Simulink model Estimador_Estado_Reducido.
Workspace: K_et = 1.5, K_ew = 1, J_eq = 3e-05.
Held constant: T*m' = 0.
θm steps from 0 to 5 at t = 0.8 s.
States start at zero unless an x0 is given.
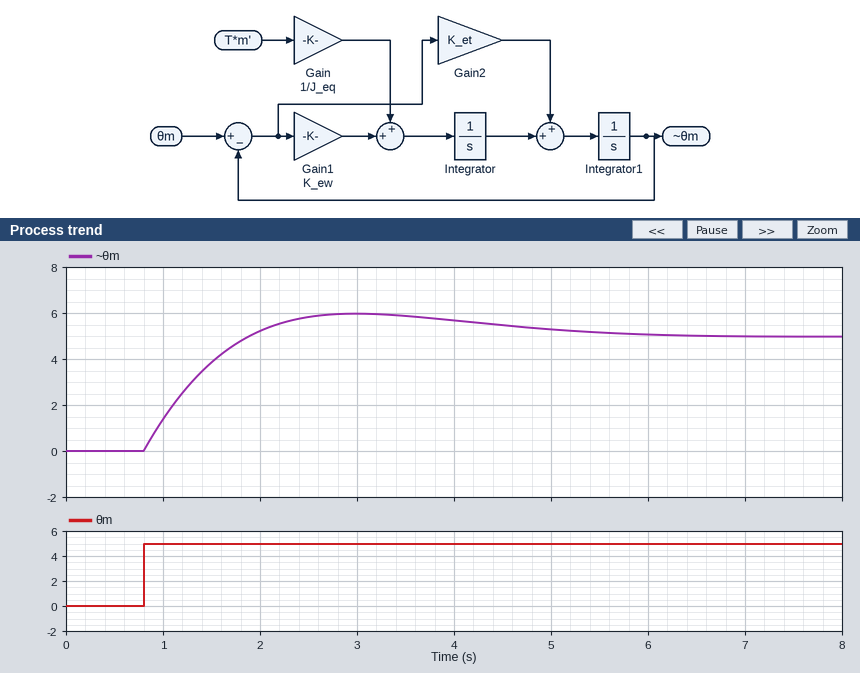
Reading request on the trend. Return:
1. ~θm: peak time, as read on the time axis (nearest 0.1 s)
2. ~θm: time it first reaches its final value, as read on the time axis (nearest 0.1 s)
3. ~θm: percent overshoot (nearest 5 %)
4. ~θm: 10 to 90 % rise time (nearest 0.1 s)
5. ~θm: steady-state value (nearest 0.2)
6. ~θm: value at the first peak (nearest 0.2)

3.0 s
1.9 s
20 %
0.8 s
5.0
6.0
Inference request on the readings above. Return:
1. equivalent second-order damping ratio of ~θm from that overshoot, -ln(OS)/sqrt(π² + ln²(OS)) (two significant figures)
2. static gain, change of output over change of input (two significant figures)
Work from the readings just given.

0.46
1.0
